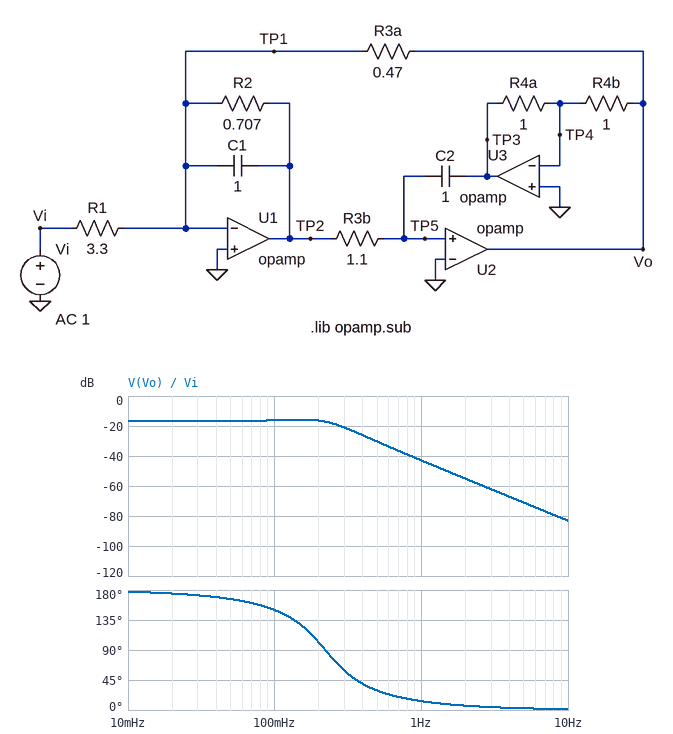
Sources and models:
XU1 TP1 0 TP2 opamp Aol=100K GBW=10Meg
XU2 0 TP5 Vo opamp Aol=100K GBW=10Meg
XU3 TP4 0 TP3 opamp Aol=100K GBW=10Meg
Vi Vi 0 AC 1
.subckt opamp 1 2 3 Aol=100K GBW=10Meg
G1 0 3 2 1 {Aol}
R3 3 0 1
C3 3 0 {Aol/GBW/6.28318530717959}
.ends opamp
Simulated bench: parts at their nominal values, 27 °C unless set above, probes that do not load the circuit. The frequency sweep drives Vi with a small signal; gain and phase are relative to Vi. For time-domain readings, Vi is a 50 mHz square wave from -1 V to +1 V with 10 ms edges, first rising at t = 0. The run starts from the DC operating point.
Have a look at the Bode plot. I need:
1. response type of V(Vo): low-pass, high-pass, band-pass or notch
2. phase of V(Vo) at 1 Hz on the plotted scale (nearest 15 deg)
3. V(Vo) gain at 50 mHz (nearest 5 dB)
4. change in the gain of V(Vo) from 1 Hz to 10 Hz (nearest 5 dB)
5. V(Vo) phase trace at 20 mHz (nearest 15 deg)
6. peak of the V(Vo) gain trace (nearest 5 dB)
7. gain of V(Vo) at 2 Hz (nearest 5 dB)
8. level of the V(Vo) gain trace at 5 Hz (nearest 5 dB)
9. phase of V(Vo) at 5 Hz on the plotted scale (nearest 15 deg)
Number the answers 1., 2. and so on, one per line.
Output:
1. low-pass
2. 15 deg
3. -15 dB
4. -40 dB
5. 180 deg
6. -15 dB
7. -55 dB
8. -70 dB
9. 0 deg
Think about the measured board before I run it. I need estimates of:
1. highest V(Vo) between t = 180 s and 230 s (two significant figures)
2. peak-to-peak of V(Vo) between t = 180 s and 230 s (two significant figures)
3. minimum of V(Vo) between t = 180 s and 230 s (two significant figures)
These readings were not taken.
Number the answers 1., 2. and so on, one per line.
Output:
1. 190 mV
2. 370 mV
3. -190 mV
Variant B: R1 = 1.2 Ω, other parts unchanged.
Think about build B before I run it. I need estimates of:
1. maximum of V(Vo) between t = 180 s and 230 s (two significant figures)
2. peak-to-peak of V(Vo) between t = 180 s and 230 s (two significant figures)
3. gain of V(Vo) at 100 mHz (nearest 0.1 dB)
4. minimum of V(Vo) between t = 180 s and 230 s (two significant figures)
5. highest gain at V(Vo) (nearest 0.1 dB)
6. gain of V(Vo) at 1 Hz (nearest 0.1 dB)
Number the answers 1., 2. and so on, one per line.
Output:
1. 510 mV
2. 1.0 V
3. -7.4 dB
4. -510 mV
5. -7.0 dB
6. -34.1 dB
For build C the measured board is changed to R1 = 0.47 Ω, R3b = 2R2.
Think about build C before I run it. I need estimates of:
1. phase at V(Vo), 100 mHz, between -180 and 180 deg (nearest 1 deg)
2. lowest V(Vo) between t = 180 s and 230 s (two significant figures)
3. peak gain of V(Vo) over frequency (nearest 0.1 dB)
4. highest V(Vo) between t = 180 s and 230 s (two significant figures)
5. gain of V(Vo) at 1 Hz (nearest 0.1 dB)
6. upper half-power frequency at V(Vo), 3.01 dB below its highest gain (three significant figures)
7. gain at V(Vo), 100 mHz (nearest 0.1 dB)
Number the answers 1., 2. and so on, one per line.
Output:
1. 123 deg
2. -1.1 V
3. 0 dB
4. 1.1 V
5. -32.2 dB
6. 154 mHz
7. -0.8 dB
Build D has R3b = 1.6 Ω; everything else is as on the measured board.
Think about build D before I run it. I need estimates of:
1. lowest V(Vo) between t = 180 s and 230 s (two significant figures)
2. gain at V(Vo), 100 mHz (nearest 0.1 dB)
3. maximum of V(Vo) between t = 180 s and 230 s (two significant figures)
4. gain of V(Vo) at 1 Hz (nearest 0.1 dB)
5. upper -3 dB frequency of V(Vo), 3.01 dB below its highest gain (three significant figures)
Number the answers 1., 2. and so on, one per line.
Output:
1. -170 mV
2. -16.7 dB
3. 170 mV
4. -46.3 dB
5. 202 mHz
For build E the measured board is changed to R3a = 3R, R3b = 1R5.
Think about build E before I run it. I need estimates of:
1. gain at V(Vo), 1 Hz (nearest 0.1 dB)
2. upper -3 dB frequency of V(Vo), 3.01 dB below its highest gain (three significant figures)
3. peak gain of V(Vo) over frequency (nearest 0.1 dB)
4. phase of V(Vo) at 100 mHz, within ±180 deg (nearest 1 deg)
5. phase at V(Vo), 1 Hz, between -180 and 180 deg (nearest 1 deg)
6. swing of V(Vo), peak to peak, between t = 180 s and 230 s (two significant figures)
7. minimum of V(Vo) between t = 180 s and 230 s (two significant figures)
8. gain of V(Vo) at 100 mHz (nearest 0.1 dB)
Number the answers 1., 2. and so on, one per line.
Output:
1. -46.0 dB
2. 28.1 mHz
3. -0.8 dB
4. 79 deg
5. 13 deg
6. 1.2 V
7. -610 mV
8. -13.0 dB
